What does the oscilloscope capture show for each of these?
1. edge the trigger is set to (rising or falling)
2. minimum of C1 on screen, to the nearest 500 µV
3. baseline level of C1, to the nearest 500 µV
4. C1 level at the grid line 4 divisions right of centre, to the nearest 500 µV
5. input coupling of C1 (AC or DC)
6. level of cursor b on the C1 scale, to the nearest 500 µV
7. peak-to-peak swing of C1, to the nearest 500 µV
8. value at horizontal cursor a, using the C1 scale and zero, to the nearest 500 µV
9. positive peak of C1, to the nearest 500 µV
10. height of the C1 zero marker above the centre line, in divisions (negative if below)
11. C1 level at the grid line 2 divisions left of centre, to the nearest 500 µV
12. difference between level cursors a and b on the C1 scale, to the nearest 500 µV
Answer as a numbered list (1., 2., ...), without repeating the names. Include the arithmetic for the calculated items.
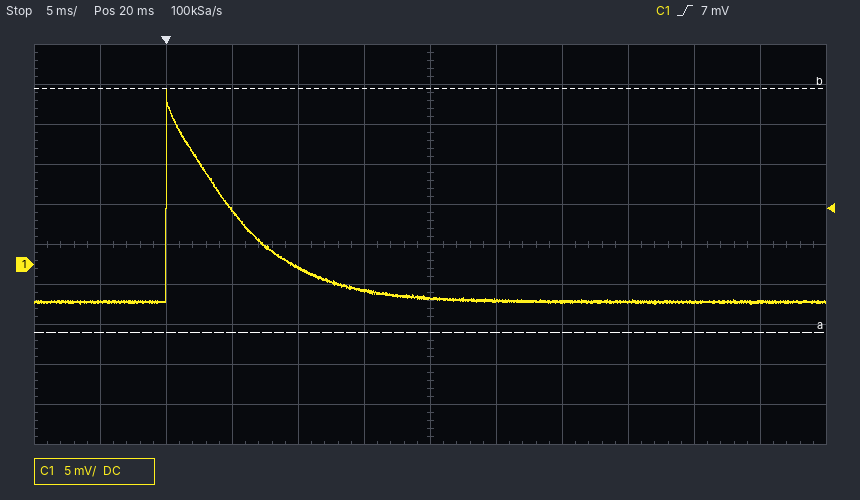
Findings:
1. rising
2. -5.0 mV
3. -4.5 mV
4. -4.5 mV
5. DC
6. 22.0 mV
7. 22.0 mV − (-5.0 mV) = 27.0 mV
8. -8.5 mV
9. 22.0 mV
10. -0.5 div
11. -500 µV
12. 30.5 mV
